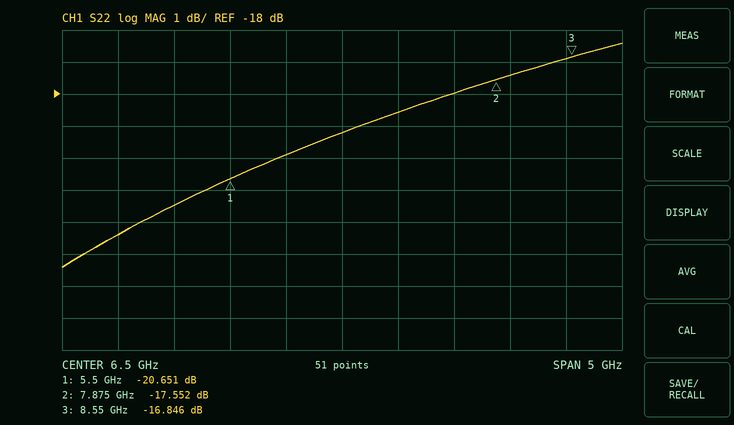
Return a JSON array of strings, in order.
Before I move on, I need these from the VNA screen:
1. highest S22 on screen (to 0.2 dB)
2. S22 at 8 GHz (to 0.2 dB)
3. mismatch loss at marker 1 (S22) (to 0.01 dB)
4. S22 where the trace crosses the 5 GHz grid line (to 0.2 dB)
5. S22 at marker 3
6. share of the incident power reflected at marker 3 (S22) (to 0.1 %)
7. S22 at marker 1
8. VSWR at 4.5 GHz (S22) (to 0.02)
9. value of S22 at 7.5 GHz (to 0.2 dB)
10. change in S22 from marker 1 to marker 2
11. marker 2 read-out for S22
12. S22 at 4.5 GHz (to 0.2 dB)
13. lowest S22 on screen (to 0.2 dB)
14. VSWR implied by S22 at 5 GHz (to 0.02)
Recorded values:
["-16.4 dB", "-17.4 dB", "0.04 dB", "-21.4 dB", "-16.846 dB", "2.1 %", "-20.651 dB", "1.16", "-18.0 dB", "3.099 dB", "-17.552 dB", "-22.4 dB", "-23.4 dB", "1.18"]
